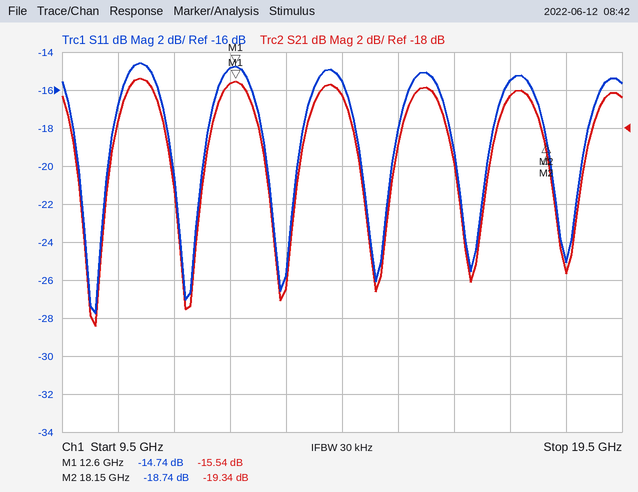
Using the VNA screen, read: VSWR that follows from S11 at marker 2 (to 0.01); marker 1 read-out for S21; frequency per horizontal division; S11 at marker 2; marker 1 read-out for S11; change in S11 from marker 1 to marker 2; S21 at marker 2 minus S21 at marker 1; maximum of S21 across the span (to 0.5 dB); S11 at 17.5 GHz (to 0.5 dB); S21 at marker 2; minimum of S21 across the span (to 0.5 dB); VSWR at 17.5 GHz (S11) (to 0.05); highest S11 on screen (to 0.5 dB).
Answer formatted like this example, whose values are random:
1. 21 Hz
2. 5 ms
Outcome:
1. 1.26
2. -15.54 dB
3. 1 GHz
4. -18.74 dB
5. -14.74 dB
6. -4.00 dB
7. -3.80 dB
8. -15.5 dB
9. -15.5 dB
10. -19.34 dB
11. -28.5 dB
12. 1.40
13. -14.5 dB
